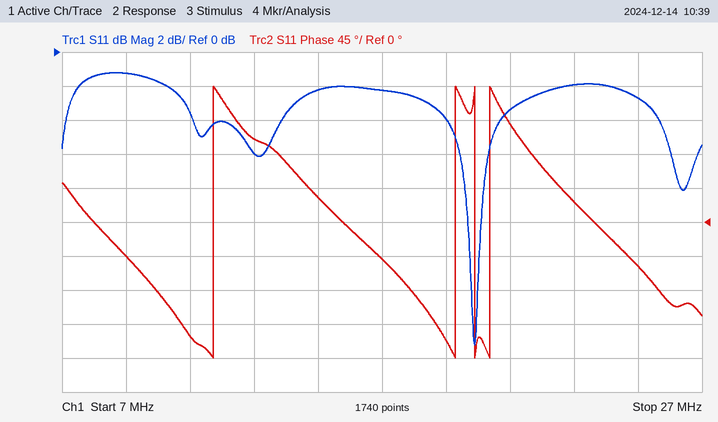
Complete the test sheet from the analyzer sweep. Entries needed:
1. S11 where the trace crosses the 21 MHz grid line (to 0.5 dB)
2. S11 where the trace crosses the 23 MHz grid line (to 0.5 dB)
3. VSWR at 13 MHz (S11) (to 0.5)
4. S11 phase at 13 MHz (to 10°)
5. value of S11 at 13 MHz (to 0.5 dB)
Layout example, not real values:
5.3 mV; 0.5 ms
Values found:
-3.5 dB; -2.0 dB; 3.0; 110°; -6.0 dB
